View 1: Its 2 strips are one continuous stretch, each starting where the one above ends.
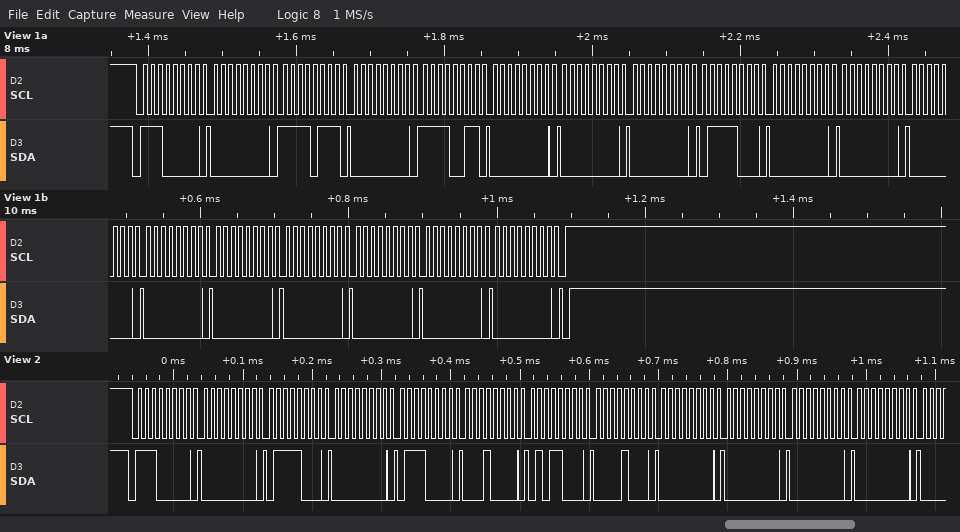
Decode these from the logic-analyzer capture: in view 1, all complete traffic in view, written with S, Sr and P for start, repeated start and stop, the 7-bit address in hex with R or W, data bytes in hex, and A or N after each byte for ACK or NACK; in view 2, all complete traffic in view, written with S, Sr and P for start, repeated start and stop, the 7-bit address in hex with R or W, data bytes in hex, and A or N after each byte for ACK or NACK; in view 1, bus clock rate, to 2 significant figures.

S 70W A 00 A F7 A 00 A F3 A 00 A 00 A 00 A 78 A 00 A 00 A 00 A 00 A 00 A 00 A 00 A 00 A 00 A P
S 70W A 00 A 78 A 00 A 70 A 10 A 58 A 08 A 00 A 00 A 00 A 00 A
100 kHz
